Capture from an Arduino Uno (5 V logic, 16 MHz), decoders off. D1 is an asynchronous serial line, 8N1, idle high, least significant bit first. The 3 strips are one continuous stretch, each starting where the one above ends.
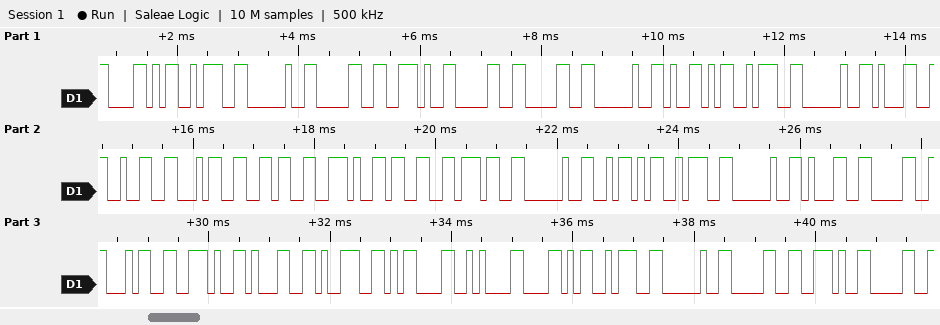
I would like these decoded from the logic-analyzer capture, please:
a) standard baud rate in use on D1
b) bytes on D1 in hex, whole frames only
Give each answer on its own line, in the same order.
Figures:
9600 baud
58 3A 20 30 2E 30 30 20 59 3A 20 31 32 34 36 2E 33 37 20 5A 3A 20 31 30 34 2E 31 39 0D 0A 58 3A 20 30 2E 30
